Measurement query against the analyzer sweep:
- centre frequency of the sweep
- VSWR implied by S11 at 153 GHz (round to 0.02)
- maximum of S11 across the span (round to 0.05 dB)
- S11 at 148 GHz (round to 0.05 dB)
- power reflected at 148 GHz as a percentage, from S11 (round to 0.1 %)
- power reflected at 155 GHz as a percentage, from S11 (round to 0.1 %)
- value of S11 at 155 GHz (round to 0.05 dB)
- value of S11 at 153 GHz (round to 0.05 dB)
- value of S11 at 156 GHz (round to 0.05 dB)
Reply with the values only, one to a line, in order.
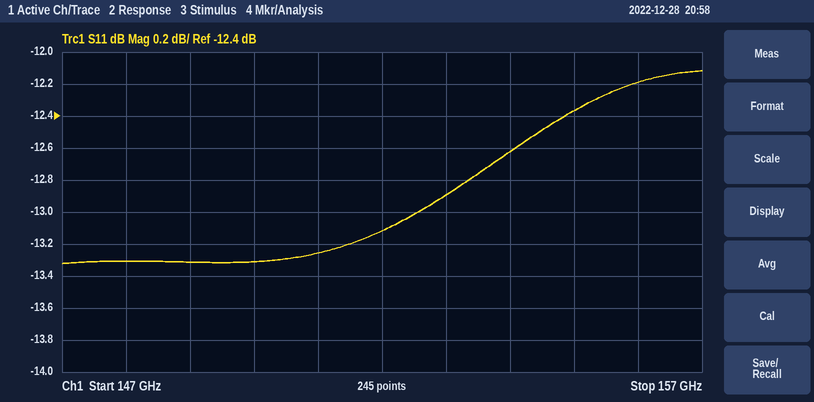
152 GHz
1.58
-12.10 dB
-13.30 dB
4.7 %
5.8 %
-12.35 dB
-12.90 dB
-12.20 dB
